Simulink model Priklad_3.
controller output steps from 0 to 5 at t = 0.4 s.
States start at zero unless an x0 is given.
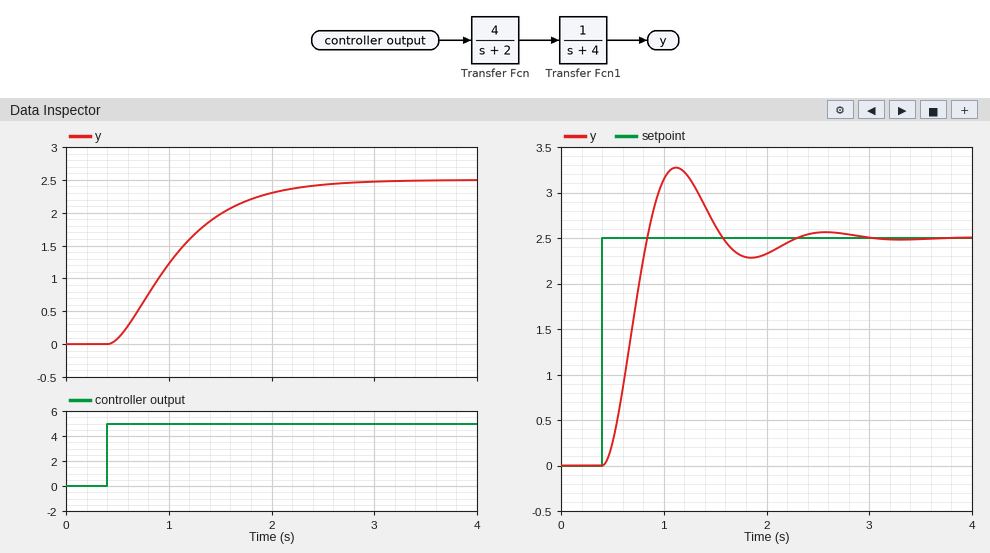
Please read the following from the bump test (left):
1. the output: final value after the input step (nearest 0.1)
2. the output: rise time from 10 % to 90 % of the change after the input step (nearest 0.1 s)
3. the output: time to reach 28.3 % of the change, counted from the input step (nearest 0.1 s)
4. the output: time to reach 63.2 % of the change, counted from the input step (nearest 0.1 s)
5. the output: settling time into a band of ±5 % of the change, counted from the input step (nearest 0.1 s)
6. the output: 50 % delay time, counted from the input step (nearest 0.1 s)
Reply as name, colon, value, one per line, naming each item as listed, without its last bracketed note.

the output: final value after the input step: 2.5
the output: rise time from 10 % to 90 % of the change after the input step: 1.3 s
the output: time to reach 28.3 % of the change, counted from the input step: 0.4 s
the output: time to reach 63.2 % of the change, counted from the input step: 0.8 s
the output: settling time into a band of ±5 % of the change, counted from the input step: 1.8 s
the output: 50 % delay time, counted from the input step: 0.6 s
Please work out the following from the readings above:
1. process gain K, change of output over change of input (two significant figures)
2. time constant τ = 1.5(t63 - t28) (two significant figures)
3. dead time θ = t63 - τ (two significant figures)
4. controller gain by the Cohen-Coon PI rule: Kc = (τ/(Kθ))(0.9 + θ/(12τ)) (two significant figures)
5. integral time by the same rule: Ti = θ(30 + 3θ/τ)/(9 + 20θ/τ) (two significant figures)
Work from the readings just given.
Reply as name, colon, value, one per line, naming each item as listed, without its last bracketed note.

process gain K, change of output over change of input: 0.50
time constant τ = 1.5(t63 - t28): 0.60 s
dead time θ = t63 - τ: 0.20 s
controller gain by the Cohen-Coon PI rule: Kc = (τ/(Kθ))(0.9 + θ/(12τ)): 5.6
integral time by the same rule: Ti = θ(30 + 3θ/τ)/(9 + 20θ/τ): 0.40 s
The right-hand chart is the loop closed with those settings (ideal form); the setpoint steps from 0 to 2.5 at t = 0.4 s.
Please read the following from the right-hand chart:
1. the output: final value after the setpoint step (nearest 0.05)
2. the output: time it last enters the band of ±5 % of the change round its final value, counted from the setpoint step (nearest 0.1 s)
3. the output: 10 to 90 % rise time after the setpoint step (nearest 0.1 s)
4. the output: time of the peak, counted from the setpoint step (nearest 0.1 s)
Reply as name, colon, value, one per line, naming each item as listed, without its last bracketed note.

the output: final value after the setpoint step: 2.50
the output: time it last enters the band of ±5 % of the change round its final value, counted from the setpoint step: 1.7 s
the output: 10 to 90 % rise time after the setpoint step: 0.3 s
the output: time of the peak, counted from the setpoint step: 0.7 s
